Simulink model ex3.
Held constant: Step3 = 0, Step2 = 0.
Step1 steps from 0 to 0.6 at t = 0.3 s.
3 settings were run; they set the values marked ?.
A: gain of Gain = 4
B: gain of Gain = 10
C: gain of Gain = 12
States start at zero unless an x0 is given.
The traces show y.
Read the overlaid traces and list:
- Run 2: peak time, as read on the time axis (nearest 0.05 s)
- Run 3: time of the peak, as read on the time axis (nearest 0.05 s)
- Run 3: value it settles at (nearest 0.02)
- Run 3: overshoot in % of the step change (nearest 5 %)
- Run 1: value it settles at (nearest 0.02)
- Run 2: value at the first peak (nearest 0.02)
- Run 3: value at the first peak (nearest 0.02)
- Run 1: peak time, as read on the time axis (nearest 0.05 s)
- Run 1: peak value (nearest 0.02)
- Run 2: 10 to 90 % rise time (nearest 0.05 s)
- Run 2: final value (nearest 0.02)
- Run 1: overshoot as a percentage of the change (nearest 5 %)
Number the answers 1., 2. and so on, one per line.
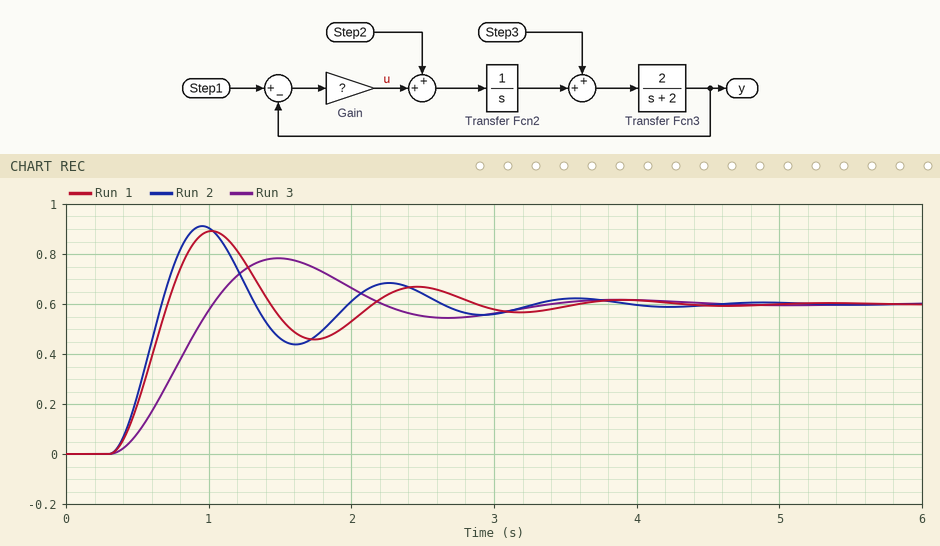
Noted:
1. 0.95 s
2. 1.50 s
3. 0.60
4. 30 %
5. 0.60
6. 0.92
7. 0.78
8. 1.00 s
9. 0.90
10. 0.25 s
11. 0.60
12. 50 %
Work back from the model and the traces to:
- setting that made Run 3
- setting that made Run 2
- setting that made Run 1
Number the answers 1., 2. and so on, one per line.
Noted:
1. A
2. C
3. B
